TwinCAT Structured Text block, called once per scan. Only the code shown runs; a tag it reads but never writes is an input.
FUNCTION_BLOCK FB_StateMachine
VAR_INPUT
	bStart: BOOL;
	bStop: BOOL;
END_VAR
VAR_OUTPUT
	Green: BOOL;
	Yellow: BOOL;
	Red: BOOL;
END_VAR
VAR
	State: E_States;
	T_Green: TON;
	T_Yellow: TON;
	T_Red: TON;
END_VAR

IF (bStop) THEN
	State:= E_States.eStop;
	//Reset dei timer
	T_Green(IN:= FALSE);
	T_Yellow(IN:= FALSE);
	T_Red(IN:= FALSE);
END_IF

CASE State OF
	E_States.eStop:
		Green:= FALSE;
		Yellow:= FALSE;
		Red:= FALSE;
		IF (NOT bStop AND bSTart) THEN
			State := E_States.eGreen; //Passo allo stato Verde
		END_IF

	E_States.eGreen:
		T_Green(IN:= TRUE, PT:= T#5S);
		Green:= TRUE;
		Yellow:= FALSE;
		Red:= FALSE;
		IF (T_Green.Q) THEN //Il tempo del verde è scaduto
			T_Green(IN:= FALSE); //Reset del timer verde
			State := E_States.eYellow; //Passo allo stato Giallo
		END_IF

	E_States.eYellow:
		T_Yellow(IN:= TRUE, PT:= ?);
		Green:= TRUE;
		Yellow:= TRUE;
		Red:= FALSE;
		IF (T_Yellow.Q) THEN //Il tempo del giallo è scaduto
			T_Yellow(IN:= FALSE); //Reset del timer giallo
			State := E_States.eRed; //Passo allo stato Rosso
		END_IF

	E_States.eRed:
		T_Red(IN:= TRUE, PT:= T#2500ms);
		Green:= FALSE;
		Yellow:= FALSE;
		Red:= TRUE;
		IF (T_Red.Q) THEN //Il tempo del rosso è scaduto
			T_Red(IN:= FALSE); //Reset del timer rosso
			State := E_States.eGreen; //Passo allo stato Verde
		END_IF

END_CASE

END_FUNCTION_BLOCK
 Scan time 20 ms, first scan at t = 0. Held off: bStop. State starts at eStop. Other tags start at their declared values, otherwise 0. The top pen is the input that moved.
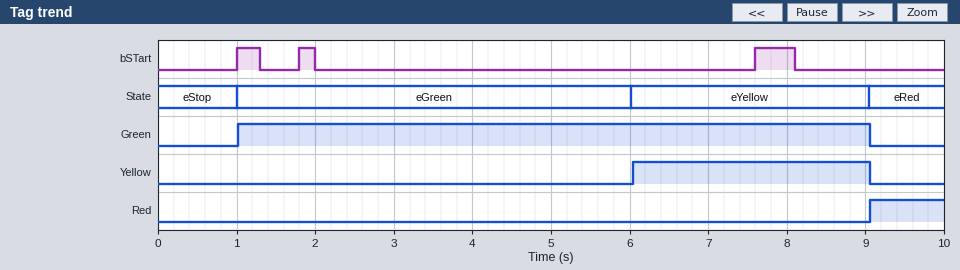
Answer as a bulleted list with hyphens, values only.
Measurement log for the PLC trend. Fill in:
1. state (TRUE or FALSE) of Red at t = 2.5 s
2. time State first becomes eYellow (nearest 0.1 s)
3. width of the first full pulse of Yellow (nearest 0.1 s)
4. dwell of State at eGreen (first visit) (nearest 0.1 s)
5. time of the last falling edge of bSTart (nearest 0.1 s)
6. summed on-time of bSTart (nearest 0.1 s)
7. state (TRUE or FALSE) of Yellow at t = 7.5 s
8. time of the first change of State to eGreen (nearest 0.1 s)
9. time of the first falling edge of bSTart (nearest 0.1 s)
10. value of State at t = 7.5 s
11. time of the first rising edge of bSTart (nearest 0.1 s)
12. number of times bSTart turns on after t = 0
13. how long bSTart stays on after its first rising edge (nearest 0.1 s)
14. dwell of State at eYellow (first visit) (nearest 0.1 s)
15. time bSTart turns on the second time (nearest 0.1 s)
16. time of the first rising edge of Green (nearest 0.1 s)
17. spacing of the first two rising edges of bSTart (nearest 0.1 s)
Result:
- FALSE
- 6.0 s
- 3.0 s
- 5.0 s
- 8.1 s
- 1.0 s
- TRUE
- 1.0 s
- 1.3 s
- eYellow
- 1.0 s
- 3
- 0.3 s
- 3.0 s
- 1.8 s
- 1.0 s
- 0.8 s
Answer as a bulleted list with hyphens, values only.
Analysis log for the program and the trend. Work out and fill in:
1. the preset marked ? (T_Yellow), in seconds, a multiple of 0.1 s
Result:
- 3.0 s
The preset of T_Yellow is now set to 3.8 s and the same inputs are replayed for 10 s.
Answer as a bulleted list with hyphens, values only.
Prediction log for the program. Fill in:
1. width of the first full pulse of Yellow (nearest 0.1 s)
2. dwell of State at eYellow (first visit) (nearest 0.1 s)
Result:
- 3.8 s
- 3.8 s
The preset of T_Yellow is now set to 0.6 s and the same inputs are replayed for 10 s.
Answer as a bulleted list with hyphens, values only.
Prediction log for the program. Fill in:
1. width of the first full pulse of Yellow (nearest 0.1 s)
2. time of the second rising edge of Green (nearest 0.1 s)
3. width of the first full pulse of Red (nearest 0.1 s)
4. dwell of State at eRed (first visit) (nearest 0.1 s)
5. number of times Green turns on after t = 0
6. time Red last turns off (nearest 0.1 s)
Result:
- 0.6 s
- 9.2 s
- 2.5 s
- 2.5 s
- 2
- 9.2 s
